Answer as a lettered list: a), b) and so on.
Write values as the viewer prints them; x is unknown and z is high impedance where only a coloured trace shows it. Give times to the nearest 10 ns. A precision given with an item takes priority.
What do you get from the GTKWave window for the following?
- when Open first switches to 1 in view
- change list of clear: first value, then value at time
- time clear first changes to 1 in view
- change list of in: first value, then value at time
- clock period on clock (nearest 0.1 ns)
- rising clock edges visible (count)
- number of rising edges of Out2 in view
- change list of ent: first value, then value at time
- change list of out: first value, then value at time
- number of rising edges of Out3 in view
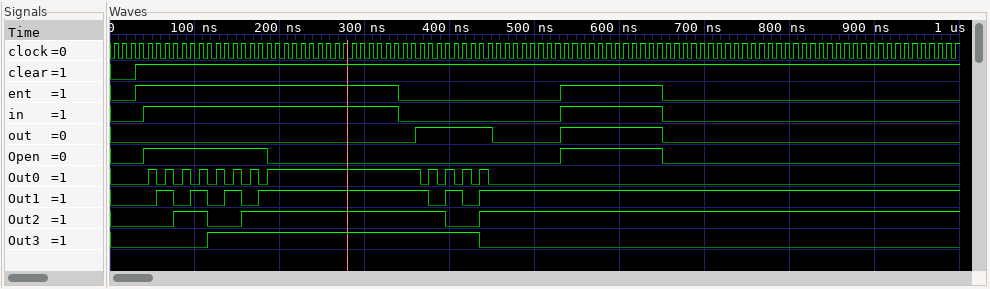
a) 40 ns
b) 0, 1 at 30 ns
c) 30 ns
d) 0, 1 at 40 ns, 0 at 340 ns, 1 at 530 ns, 0 at 650 ns
e) 10 ns
f) 100
g) 3
h) 0, 1 at 30 ns, 0 at 340 ns, 1 at 530 ns, 0 at 650 ns
i) 0, 1 at 360 ns, 0 at 450 ns, 1 at 530 ns, 0 at 650 ns
j) 1
